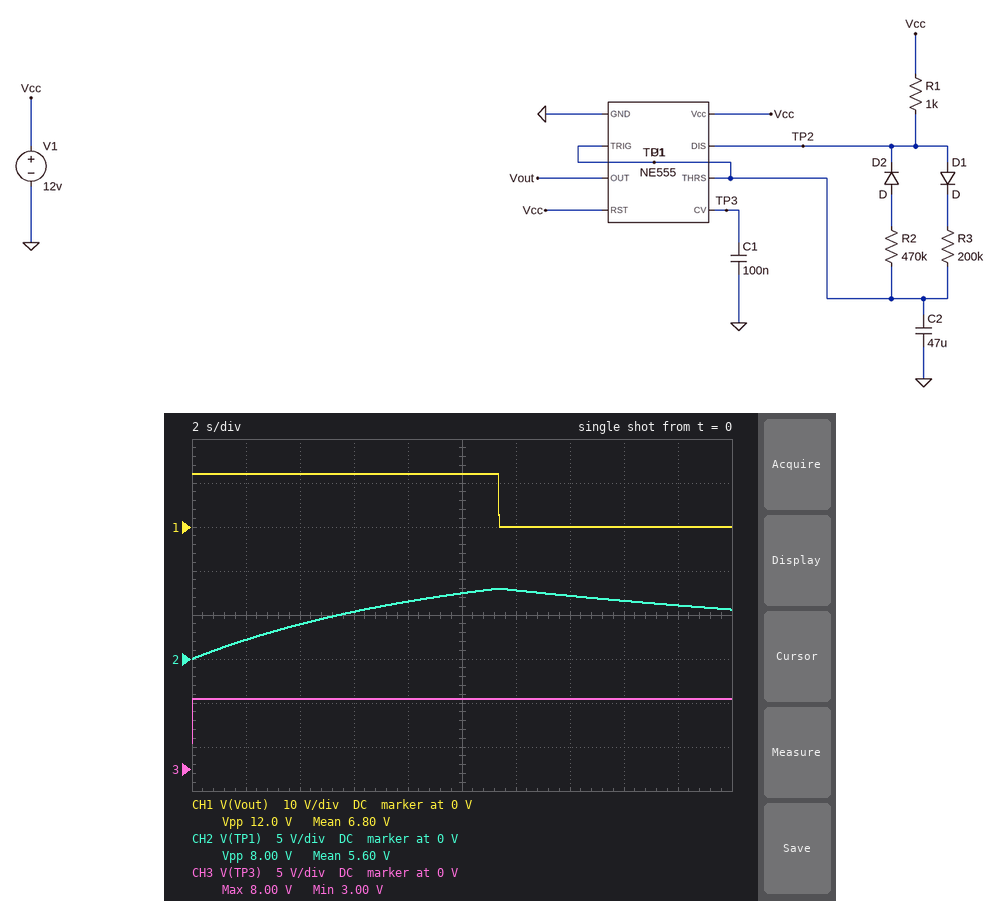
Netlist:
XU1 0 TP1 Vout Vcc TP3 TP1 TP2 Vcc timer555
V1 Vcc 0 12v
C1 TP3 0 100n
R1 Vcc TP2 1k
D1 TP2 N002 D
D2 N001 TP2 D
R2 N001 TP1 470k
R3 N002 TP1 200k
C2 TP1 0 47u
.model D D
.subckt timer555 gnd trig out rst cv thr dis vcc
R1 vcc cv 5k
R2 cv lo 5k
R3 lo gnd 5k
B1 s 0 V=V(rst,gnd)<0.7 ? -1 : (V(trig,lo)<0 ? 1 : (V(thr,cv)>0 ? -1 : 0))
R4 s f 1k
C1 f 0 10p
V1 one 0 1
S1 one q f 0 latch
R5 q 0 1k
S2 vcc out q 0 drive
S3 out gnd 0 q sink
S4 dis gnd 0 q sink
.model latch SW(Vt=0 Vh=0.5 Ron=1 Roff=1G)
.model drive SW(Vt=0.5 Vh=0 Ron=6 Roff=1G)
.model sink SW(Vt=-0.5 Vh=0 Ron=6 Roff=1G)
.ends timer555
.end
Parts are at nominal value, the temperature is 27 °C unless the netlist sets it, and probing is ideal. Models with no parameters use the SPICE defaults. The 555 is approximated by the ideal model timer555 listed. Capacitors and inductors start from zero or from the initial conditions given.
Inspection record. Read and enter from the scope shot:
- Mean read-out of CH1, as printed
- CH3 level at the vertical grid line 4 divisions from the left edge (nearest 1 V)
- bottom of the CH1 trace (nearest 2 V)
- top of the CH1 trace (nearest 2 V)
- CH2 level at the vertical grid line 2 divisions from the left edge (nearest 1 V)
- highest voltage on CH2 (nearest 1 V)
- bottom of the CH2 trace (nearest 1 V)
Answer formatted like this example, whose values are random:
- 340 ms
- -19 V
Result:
- 6.80 V
- 8 V
- 0 V
- 12 V
- 4 V
- 8 V
- 0 V
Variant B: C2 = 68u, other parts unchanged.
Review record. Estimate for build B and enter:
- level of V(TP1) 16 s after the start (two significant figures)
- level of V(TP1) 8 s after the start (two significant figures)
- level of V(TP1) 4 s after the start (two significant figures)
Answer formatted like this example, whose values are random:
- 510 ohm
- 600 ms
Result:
- 7.9 V
- 5.1 V
- 2.9 V
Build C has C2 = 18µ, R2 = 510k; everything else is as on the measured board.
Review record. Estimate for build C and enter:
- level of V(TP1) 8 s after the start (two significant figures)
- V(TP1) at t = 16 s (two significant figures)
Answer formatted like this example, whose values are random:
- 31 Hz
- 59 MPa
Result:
- 5.6 V
- 6.7 V
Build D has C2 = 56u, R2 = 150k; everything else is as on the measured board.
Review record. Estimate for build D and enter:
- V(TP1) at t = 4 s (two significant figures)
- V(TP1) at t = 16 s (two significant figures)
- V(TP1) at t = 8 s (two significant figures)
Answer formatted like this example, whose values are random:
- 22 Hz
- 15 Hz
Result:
- 3.4 V
- 6.1 V
- 5.8 V
